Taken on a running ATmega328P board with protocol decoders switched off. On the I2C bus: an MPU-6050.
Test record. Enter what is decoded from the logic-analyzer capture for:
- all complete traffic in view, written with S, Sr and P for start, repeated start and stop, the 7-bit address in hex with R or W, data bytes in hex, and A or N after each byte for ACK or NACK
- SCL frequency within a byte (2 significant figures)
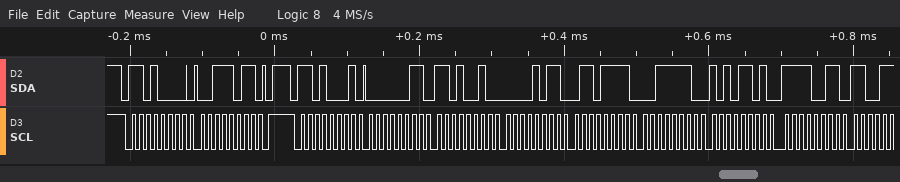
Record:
S 68W A 3B A P S 68R A 03 A D2 A 0B A 6F A 3E A AD A F3 A
100 kHz
